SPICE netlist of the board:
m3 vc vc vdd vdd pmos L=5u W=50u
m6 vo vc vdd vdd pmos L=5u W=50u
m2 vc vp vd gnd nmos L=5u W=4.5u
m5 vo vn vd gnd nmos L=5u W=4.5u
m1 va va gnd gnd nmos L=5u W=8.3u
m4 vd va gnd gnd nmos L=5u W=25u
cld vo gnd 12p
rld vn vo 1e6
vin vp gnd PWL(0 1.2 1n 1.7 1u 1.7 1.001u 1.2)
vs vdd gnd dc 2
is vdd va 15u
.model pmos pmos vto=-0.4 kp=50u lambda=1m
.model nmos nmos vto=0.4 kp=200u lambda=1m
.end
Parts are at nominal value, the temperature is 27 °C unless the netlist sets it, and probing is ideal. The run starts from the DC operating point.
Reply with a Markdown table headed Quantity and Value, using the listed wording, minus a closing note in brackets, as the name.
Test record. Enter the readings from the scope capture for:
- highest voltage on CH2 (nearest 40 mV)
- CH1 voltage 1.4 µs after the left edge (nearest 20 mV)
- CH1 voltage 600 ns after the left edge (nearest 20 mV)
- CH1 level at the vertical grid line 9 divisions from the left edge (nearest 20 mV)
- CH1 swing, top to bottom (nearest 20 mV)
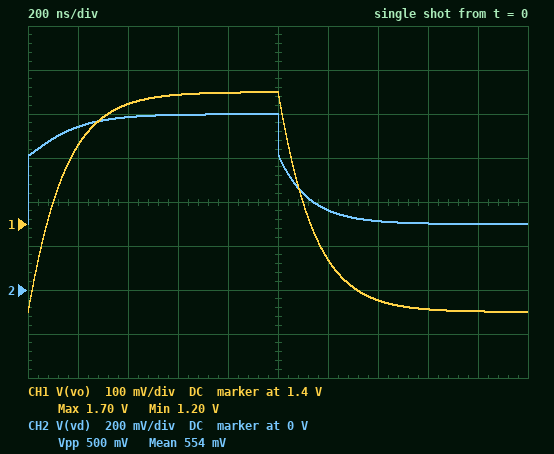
| Quantity | Value |
|---|---|
| highest voltage on CH2 | 800 mV |
| CH1 voltage 1.4 µs after the left edge | 1.22 V |
| CH1 voltage 600 ns after the left edge | 1.70 V |
| CH1 level at the vertical grid line 9 divisions from the left edge | 1.20 V |
| CH1 swing, top to bottom | 500 mV |
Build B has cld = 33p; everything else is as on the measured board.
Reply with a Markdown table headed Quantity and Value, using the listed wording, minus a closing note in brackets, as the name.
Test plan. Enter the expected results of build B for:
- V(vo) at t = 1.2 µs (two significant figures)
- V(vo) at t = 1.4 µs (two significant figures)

| Quantity | Value |
|---|---|
| V(vo) at t = 1.2 µs | 1.5 V |
| V(vo) at t = 1.4 µs | 1.4 V |
